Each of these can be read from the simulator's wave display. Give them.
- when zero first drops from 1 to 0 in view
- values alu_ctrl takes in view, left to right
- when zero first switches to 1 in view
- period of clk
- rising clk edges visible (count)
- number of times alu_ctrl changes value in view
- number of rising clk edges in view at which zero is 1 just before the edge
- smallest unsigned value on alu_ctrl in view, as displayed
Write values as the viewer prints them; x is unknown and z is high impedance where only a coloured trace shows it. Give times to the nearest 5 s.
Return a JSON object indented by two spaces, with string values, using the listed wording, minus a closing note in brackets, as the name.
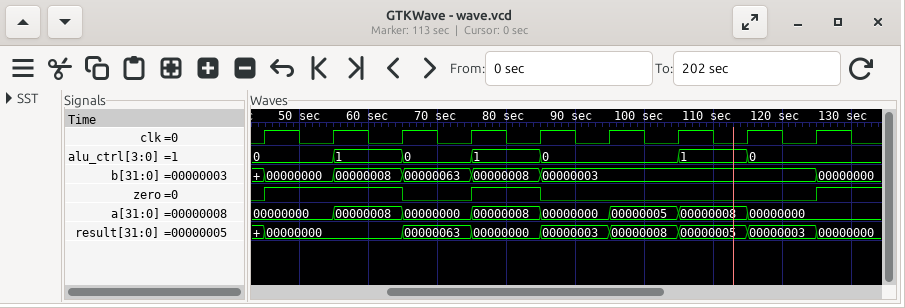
{
  "when zero first drops from 1 to 0 in view": "65 s",
  "values alu_ctrl takes in view, left to right": "0, 1, 0, 1, 0, 1, 0",
  "when zero first switches to 1 in view": "45 s",
  "period of clk": "10 s",
  "rising clk edges visible": "9",
  "number of times alu_ctrl changes value in view": "6",
  "number of rising clk edges in view at which zero is 1 just before the edge": "3",
  "smallest unsigned value on alu_ctrl in view, as displayed": "0"
}
